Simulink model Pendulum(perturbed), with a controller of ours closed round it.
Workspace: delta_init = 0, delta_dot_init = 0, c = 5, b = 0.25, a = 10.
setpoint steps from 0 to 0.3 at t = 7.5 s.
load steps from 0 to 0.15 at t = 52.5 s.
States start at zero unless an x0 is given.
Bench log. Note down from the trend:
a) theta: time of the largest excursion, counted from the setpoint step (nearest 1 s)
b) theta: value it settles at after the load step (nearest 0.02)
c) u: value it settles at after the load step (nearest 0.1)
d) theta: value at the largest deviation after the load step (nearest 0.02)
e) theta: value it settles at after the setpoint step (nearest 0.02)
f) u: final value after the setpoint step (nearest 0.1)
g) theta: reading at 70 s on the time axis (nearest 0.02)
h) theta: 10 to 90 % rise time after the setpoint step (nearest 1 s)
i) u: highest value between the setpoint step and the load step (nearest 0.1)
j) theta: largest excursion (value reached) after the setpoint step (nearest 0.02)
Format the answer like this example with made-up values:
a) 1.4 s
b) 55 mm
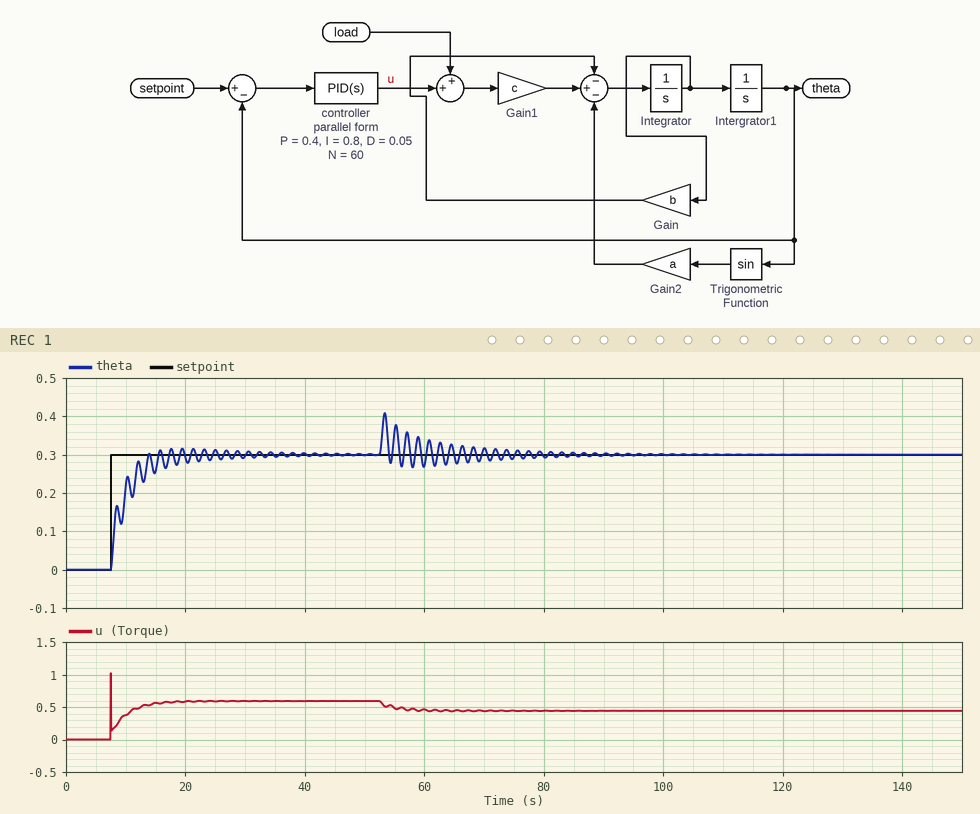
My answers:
a) 12 s
b) 0.30
c) 0.4
d) 0.40
e) 0.30
f) 0.6
g) 0.32
h) 4 s
i) 1.0
j) 0.32
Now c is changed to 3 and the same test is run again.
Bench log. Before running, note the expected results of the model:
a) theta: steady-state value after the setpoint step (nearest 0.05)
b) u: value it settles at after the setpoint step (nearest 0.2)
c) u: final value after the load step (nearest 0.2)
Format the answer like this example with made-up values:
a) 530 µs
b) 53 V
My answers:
a) 0.30
b) 1.0
c) 0.8
